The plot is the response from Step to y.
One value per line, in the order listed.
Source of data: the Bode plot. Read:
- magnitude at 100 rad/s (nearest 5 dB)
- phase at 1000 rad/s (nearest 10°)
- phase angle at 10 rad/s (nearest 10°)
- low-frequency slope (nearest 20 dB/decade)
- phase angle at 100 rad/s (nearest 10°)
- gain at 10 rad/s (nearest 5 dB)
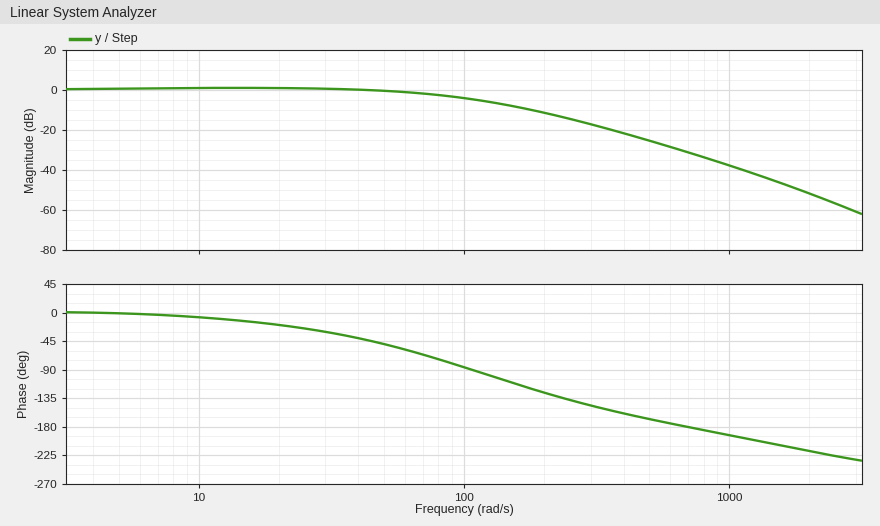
-5 dB
-190°
-10°
0 dB/decade
-90°
0 dB
